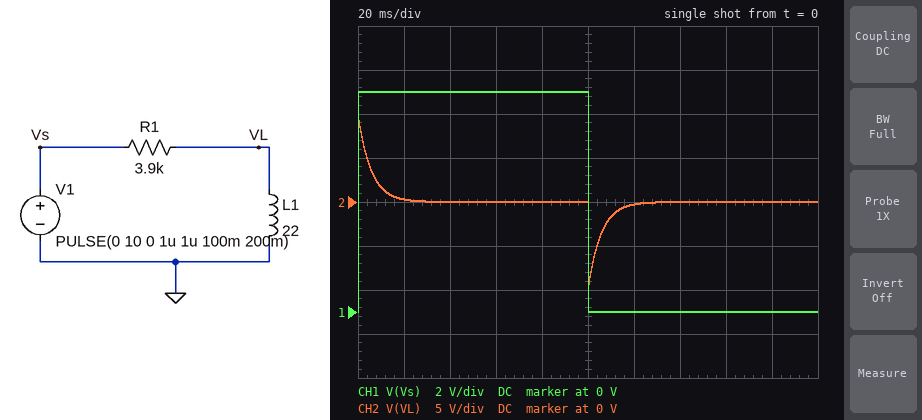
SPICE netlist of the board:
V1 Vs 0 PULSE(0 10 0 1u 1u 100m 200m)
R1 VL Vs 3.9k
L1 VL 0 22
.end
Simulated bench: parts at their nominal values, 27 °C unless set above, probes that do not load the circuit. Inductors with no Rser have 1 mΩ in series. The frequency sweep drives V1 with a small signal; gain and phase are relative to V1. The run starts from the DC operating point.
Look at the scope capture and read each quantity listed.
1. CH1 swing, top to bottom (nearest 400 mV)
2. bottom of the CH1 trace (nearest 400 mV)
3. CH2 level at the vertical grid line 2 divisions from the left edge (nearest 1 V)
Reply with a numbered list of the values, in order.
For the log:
1. 10.0 V
2. 0 V
3. 0 V
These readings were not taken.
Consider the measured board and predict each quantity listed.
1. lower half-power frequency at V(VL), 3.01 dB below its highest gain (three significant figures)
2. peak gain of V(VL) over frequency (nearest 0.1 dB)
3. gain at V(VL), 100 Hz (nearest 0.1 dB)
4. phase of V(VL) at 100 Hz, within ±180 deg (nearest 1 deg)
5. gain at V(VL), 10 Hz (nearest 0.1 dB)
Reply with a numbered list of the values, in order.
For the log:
1. 28.2 Hz
2. 0 dB
3. -0.3 dB
4. 16 deg
5. -9.5 dB
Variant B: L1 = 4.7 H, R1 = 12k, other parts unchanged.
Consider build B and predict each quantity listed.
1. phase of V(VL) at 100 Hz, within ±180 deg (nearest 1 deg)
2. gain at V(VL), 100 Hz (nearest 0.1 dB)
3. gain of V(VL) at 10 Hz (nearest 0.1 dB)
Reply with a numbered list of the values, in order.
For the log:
1. 76 deg
2. -12.4 dB
3. -32.2 dB
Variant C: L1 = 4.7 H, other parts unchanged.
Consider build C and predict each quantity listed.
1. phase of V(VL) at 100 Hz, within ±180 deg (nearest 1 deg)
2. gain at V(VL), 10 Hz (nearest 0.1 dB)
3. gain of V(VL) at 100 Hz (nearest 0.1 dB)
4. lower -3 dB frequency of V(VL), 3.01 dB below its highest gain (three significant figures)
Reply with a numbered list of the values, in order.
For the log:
1. 53 deg
2. -22.4 dB
3. -4.4 dB
4. 132 Hz
